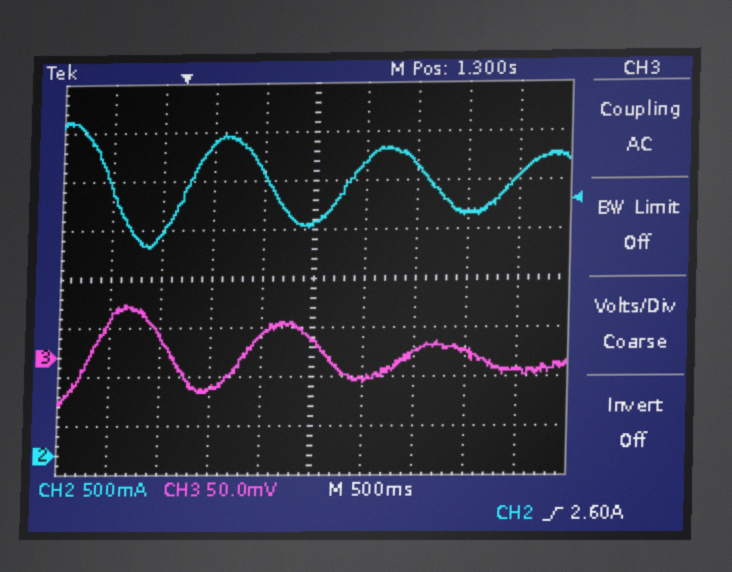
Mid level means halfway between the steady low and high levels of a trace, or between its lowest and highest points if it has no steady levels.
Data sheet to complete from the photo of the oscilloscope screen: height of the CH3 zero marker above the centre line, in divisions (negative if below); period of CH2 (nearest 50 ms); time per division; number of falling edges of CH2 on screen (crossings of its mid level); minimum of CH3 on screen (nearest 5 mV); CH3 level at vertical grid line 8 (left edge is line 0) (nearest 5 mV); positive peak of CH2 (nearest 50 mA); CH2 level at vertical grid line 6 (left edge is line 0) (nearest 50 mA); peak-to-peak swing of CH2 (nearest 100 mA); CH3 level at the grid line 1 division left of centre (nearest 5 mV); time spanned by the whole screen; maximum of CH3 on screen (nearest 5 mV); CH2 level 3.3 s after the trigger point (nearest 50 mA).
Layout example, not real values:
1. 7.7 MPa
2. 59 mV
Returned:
1. -1.6 div
2. 1.60 s
3. 500 ms
4. 3
5. -50 mV
6. 5 mV
7. 3.40 A
8. 3.00 A
9. 1.30 A
10. 20 mV
11. 5 s
12. 55 mV
13. 2.85 A
